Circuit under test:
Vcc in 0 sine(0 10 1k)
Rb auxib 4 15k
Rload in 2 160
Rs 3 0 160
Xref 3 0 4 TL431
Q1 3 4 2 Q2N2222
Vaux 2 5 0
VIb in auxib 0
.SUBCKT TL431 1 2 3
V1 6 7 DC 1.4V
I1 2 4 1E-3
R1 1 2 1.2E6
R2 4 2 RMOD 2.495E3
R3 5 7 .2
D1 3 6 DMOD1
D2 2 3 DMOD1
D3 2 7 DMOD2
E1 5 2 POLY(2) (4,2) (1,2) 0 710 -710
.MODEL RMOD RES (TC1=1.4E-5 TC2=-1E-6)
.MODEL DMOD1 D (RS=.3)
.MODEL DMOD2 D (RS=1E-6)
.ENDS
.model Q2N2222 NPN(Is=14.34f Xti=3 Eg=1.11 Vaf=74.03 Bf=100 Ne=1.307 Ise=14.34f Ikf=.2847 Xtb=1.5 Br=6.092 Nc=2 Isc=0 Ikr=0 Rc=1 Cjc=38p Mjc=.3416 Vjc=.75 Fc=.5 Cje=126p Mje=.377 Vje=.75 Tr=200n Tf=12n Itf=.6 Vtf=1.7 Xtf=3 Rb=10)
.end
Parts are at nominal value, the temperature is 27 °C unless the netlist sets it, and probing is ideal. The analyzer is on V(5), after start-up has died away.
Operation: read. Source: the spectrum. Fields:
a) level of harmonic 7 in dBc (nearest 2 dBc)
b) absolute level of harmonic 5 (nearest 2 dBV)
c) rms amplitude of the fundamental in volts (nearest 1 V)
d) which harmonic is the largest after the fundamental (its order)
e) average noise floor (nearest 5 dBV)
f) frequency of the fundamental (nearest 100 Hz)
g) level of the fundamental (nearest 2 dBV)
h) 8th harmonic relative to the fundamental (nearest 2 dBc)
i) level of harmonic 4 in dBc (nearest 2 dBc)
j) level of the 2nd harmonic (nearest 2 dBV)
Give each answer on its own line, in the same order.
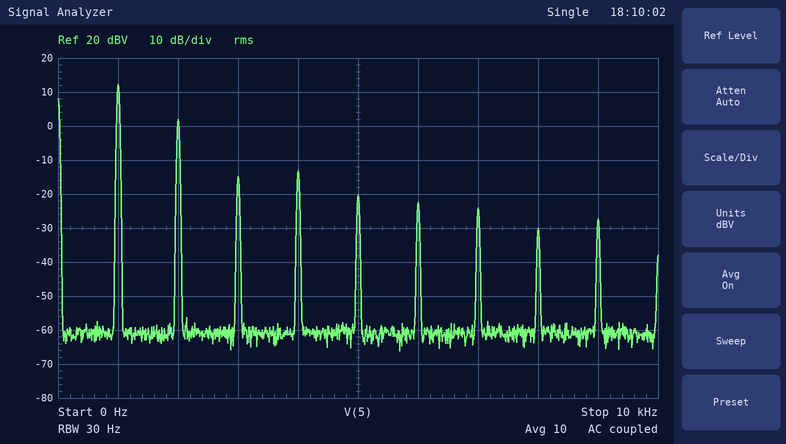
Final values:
-36 dBc
-20 dBV
4 V
2
-60 dBV
1.0 kHz
12 dBV
-42 dBc
-26 dBc
2 dBV
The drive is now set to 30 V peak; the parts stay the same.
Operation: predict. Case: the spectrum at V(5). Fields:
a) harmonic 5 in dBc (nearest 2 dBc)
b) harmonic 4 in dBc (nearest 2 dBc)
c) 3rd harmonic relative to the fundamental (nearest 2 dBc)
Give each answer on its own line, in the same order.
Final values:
-40 dBc
-24 dBc
-34 dBc
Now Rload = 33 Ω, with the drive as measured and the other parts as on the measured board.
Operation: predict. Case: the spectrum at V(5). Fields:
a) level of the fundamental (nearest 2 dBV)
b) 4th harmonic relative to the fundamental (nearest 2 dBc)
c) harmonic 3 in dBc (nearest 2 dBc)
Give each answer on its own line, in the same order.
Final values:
14 dBV
-28 dBc
-30 dBc
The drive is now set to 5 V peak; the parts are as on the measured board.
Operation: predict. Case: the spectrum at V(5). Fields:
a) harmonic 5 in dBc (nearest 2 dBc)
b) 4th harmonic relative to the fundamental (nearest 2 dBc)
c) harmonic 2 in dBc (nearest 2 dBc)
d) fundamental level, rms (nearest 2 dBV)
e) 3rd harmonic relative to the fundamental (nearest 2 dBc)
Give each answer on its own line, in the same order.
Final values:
-30 dBc
-30 dBc
-12 dBc
8 dBV
-24 dBc
